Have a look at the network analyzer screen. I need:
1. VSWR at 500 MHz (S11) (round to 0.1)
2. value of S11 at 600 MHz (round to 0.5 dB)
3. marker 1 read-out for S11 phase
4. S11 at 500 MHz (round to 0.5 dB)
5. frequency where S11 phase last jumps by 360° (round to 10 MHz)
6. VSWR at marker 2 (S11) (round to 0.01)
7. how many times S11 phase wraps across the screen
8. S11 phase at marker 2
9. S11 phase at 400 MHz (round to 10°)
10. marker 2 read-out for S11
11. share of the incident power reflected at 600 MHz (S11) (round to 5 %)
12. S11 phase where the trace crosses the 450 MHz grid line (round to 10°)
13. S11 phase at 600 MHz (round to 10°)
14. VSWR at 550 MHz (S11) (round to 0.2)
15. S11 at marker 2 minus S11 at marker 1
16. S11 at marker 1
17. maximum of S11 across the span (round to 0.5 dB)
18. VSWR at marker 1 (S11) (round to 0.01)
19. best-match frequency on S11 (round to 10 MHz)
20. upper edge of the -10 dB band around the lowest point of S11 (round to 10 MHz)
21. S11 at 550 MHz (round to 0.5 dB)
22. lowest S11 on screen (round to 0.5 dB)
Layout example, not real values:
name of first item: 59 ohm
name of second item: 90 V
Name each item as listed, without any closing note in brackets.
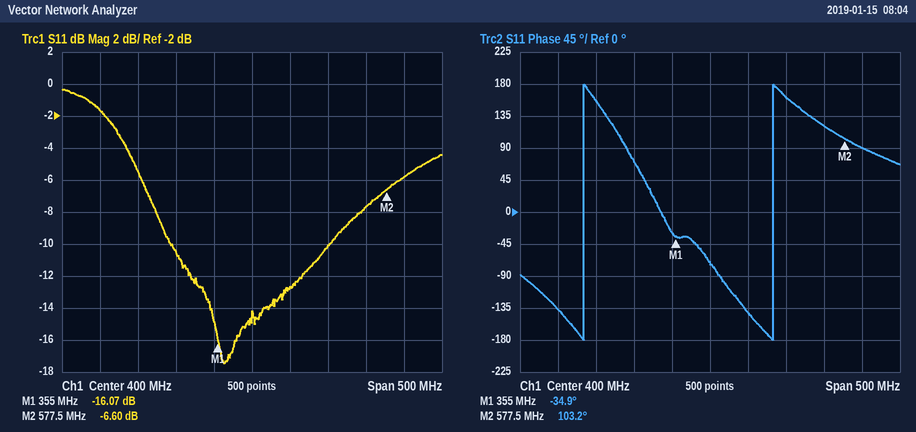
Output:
VSWR at 500 MHz (S11): 1.9
value of S11 at 600 MHz: -6.0 dB
marker 1 read-out for S11 phase: -34.9°
S11 at 500 MHz: -10.0 dB
frequency where S11 phase last jumps by 360°: 480 MHz
VSWR at marker 2 (S11): 2.76
how many times S11 phase wraps across the screen: 2
S11 phase at marker 2: 103.2°
S11 phase at 400 MHz: -70°
marker 2 read-out for S11: -6.60 dB
share of the incident power reflected at 600 MHz (S11): 25 %
S11 phase where the trace crosses the 450 MHz grid line: -140°
S11 phase at 600 MHz: 90°
VSWR at 550 MHz (S11): 2.4
S11 at marker 2 minus S11 at marker 1: 9.47 dB
S11 at marker 1: -16.07 dB
maximum of S11 across the span: -0.5 dB
VSWR at marker 1 (S11): 1.37
best-match frequency on S11: 360 MHz
upper edge of the -10 dB band around the lowest point of S11: 500 MHz
S11 at 550 MHz: -7.5 dB
lowest S11 on screen: -17.5 dB
